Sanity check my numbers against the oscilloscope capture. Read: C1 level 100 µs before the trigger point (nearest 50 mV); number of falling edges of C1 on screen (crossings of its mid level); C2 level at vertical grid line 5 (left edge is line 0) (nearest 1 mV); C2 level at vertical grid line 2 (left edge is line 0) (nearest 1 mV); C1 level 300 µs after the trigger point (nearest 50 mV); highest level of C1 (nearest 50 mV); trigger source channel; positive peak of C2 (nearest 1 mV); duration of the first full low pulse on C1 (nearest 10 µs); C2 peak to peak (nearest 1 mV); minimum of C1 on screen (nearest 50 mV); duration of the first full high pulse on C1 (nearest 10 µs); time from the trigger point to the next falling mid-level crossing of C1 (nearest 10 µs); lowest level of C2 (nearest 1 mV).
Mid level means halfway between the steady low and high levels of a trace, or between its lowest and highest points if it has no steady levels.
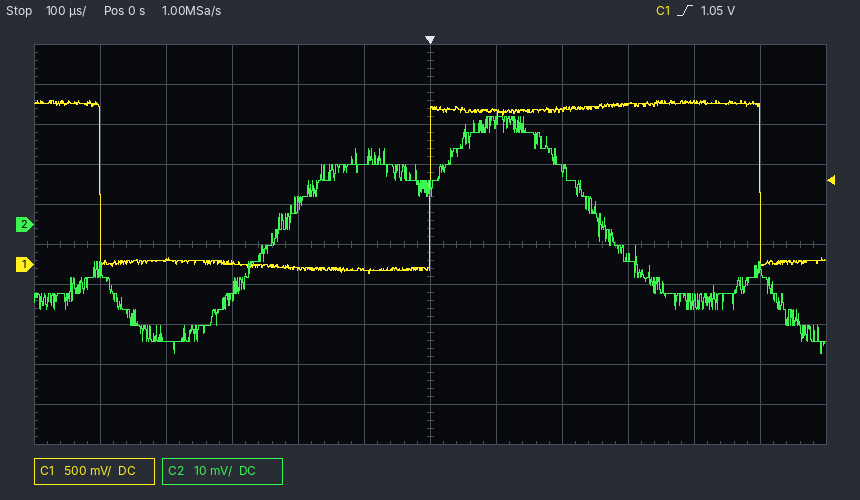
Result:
-50 mV
2
15 mV
-29 mV
2.00 V
2.05 V
C1
27 mV
500 µs
59 mV
-100 mV
500 µs
500 µs
-32 mV
